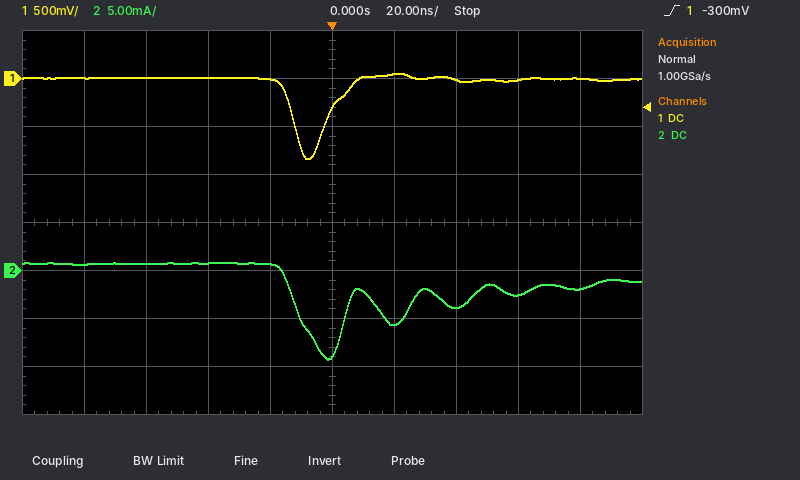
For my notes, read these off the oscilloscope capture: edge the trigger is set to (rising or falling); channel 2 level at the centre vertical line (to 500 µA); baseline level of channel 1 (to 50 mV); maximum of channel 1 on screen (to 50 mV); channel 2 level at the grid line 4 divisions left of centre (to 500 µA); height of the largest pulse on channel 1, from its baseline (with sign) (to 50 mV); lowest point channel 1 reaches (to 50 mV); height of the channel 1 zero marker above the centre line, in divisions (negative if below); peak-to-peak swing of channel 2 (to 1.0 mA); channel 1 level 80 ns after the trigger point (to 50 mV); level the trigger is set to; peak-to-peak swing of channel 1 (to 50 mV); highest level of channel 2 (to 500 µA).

rising
-9.0 mA
0 mV
50 mV
500 µA
-850 mV
-850 mV
+3.0 div
10.0 mA
0 mV
-300 mV
900 mV
1.0 mA
